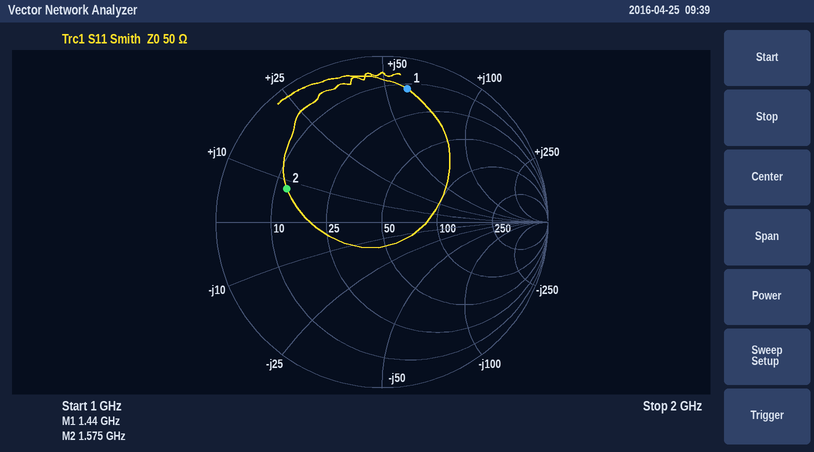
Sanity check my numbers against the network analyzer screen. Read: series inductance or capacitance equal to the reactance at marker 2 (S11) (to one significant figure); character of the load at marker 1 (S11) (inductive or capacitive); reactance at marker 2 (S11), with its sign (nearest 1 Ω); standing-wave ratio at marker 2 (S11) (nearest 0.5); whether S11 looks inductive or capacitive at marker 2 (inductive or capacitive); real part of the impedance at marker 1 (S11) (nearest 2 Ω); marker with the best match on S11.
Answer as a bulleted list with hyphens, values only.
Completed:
- 800 pH
- inductive
- +8 Ω
- 4.0
- inductive
- 12 Ω
- marker 2
